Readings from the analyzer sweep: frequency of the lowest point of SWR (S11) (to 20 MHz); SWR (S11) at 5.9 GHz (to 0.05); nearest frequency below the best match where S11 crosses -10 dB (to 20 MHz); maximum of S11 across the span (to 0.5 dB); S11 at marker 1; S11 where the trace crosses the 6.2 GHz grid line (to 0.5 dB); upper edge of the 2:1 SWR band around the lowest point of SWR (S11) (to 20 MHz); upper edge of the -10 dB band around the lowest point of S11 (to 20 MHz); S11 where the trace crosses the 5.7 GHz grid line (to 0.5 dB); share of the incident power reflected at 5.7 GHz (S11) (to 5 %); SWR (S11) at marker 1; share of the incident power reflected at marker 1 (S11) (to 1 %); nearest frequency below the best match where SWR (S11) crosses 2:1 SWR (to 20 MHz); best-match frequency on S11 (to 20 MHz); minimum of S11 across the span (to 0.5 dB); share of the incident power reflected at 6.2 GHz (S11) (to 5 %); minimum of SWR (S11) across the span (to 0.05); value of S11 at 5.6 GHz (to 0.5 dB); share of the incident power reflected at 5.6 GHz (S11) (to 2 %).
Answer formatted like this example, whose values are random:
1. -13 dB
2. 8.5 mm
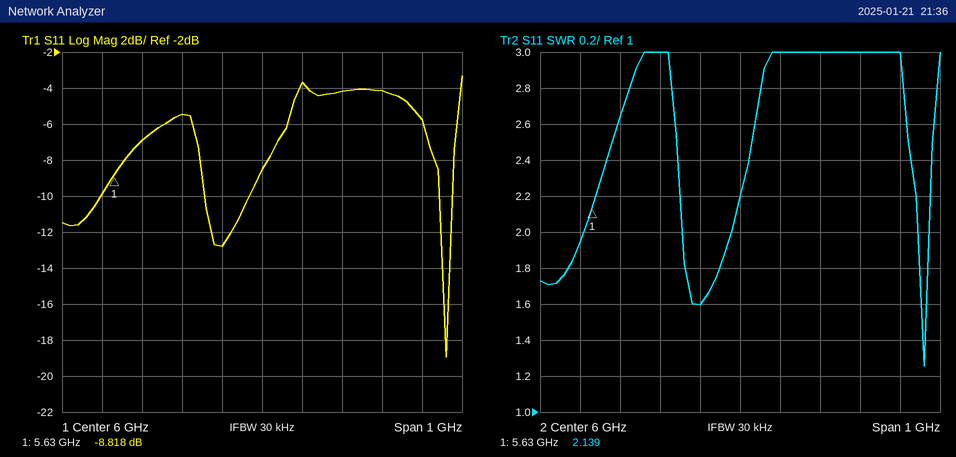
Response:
1. 6.46 GHz
2. 1.60
3. 6.44 GHz
4. -3.5 dB
5. -8.818 dB
6. -4.0 dB
7. 6.48 GHz
8. 6.48 GHz
9. -7.0 dB
10. 20 %
11. 2.139
12. 13 %
13. 6.44 GHz
14. 6.46 GHz
15. -19.0 dB
16. 40 %
17. 1.25
18. -10.0 dB
19. 10 %
